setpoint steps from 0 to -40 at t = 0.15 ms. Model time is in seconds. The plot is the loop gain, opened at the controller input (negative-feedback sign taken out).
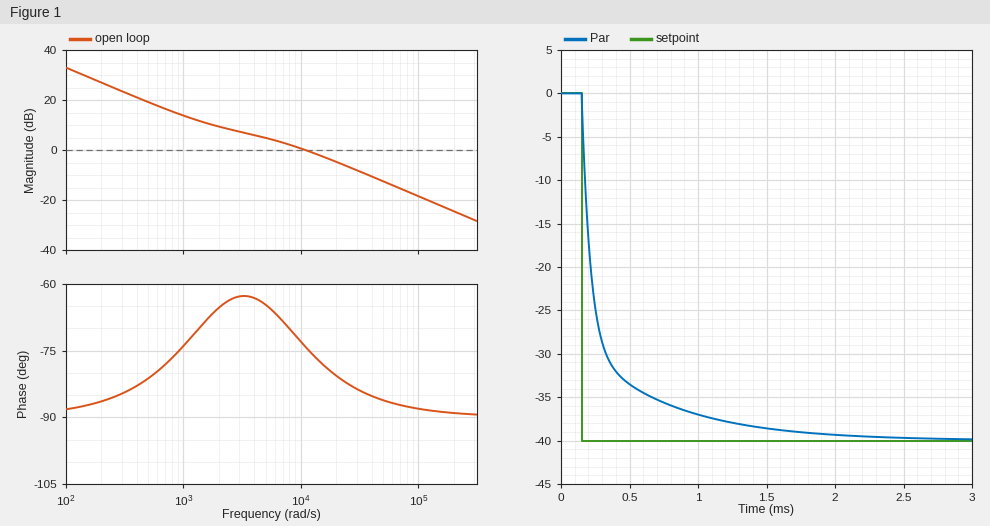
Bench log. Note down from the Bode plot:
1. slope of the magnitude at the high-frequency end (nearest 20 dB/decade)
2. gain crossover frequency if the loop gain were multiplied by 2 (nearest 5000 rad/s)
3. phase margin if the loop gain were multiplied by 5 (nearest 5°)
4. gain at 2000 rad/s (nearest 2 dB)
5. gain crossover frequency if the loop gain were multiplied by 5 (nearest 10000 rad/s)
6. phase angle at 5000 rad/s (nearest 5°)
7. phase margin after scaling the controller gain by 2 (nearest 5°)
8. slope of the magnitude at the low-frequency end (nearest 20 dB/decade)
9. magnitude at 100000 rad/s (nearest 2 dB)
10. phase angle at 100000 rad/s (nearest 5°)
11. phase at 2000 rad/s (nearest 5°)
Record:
-20 dB/decade
25000 rad/s
95°
10 dB
60000 rad/s
-65°
100°
-20 dB/decade
-18 dB
-90°
-65°
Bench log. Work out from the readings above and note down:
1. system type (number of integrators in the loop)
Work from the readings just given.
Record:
1
